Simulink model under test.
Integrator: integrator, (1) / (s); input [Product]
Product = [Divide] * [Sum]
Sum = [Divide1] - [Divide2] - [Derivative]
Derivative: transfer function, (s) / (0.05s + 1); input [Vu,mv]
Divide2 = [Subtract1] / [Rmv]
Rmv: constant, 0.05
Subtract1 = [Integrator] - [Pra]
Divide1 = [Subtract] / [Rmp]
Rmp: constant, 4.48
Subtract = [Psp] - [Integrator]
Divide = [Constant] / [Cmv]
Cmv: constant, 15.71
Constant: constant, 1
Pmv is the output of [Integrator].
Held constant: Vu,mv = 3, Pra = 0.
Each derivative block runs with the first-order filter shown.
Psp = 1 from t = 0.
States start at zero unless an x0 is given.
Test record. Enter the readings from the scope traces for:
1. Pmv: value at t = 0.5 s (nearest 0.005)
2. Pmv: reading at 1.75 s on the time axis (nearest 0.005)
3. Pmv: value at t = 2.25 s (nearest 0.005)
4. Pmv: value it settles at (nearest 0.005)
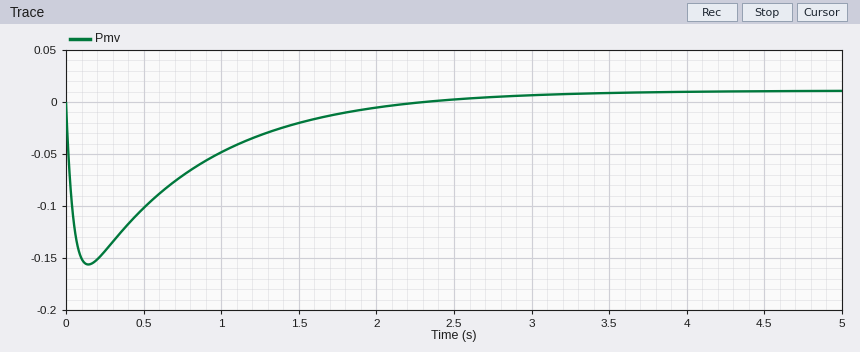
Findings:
-0.100
-0.010
0.000
0.010
